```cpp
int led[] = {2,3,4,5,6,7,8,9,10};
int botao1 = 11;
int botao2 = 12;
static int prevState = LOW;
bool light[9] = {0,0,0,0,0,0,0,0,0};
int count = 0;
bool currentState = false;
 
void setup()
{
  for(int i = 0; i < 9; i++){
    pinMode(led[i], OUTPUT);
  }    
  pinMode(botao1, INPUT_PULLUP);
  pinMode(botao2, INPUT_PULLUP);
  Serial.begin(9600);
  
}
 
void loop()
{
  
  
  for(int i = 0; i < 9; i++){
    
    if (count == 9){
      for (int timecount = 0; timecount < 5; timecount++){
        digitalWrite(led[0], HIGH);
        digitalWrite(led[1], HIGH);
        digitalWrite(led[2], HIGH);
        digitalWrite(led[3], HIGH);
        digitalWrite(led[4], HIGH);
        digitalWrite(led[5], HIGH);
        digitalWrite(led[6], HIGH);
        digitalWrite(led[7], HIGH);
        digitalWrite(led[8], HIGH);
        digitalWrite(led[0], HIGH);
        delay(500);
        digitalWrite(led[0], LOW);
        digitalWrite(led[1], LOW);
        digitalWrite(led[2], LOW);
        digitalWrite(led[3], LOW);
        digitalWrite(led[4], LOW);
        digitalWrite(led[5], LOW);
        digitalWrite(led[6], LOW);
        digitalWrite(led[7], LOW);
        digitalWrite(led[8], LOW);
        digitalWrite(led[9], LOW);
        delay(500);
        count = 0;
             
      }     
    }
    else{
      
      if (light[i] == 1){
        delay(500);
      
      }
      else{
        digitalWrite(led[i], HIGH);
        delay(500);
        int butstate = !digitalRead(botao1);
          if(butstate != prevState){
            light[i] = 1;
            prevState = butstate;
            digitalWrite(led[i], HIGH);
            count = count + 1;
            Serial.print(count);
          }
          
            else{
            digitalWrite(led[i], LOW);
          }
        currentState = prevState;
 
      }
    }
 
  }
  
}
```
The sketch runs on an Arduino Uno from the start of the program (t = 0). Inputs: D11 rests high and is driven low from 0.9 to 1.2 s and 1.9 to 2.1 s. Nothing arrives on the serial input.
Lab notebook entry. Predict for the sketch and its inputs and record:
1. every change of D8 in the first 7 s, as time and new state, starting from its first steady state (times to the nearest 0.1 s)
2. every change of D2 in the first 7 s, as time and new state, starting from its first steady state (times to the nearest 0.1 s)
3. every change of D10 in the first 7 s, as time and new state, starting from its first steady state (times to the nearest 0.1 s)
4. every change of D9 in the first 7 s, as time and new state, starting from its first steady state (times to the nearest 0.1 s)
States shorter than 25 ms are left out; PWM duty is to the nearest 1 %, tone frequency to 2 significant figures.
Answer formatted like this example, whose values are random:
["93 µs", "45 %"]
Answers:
["0 s low; 3 s high; 3.5 s low", "0 s high; 0.5 s low; 4.5 s high; 5 s low", "0 s low; 4 s high; 4.5 s low", "0 s low; 3.5 s high; 4 s low"]
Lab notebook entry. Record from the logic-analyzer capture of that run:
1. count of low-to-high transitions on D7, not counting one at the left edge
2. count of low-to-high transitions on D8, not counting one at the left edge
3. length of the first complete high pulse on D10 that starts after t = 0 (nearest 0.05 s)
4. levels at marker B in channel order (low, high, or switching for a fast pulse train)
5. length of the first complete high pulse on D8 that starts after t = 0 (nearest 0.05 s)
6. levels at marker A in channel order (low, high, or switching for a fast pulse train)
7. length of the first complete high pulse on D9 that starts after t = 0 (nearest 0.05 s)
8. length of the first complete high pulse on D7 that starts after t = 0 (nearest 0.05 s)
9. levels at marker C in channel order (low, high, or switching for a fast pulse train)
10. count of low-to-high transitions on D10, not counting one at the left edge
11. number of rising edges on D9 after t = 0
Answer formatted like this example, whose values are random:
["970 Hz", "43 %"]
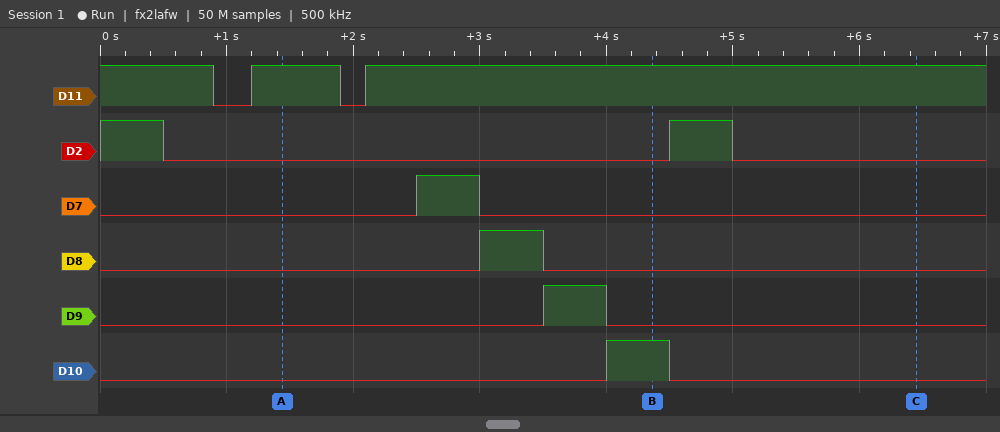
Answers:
["1", "1", "0.50 s", "D11 high, D2 low, D7 low, D8 low, D9 low, D10 high", "0.50 s", "D11 high, D2 low, D7 low, D8 low, D9 low, D10 low", "0.50 s", "0.50 s", "D11 high, D2 low, D7 low, D8 low, D9 low, D10 low", "1", "1"]
